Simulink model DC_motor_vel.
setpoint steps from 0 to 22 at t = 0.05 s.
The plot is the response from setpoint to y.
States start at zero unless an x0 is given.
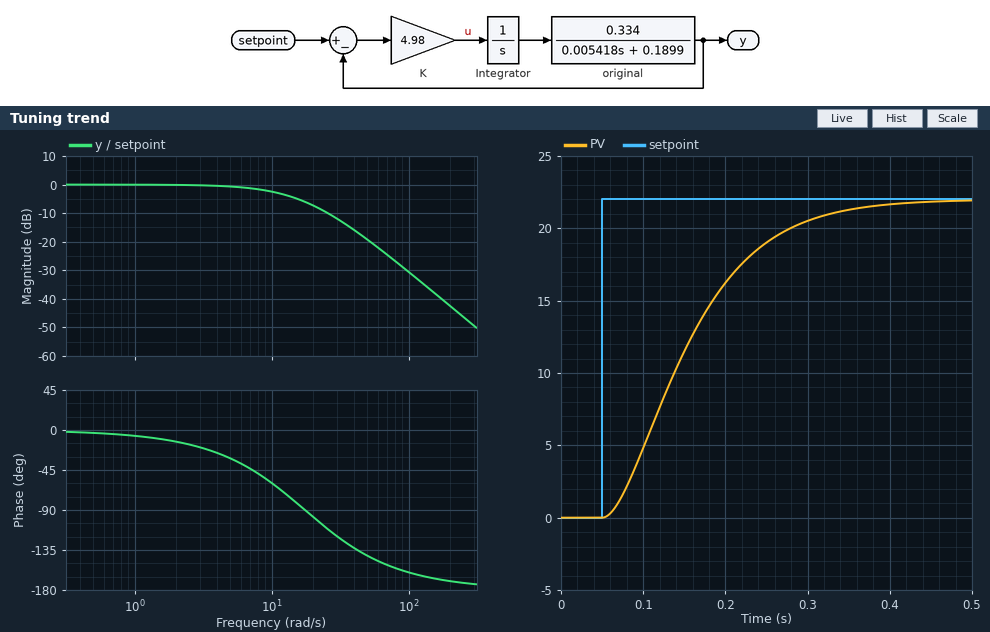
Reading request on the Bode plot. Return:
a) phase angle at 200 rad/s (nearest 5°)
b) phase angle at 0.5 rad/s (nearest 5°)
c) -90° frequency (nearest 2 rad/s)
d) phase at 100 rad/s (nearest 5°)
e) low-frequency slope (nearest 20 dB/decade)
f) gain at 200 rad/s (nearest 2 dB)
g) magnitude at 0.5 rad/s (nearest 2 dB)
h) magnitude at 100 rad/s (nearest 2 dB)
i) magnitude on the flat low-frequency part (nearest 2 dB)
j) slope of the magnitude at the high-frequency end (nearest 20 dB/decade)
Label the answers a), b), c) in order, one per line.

a) -170°
b) -5°
c) 18 rad/s
d) -160°
e) 0 dB/decade
f) -42 dB
g) 0 dB
h) -30 dB
i) 0 dB
j) -40 dB/decade
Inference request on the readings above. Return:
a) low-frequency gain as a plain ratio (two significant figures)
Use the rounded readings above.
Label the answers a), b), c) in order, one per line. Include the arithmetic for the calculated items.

a) 10^(0 / 20) = 1.0
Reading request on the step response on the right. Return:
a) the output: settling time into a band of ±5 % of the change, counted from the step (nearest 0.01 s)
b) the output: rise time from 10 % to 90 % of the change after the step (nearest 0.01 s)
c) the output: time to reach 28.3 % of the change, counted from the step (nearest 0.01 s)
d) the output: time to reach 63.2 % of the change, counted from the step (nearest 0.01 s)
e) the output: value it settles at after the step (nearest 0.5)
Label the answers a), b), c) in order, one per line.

a) 0.27 s
b) 0.19 s
c) 0.06 s
d) 0.12 s
e) 22.0
